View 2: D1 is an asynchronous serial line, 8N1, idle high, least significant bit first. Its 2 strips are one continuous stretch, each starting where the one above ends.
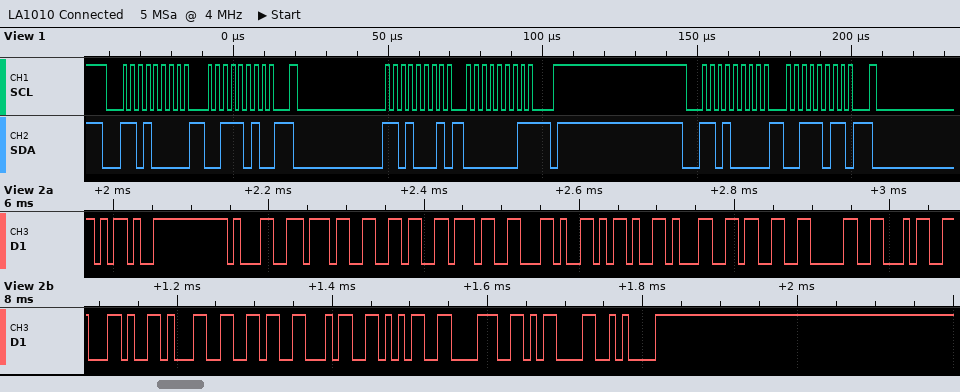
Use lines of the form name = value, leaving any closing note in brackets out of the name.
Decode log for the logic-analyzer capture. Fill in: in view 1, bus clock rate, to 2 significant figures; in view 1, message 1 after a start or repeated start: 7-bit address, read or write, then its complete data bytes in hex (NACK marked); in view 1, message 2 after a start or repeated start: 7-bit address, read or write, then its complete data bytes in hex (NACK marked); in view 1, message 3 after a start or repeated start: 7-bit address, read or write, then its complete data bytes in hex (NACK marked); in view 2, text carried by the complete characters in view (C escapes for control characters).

in view 1, bus clock rate, to 2 significant figures = 400 kHz
in view 1, message 1 after a start or repeated start: 7-bit address, read or write, then its complete data bytes in hex = 0x68 write: 3A
in view 1, message 2 after a start or repeated start: 7-bit address, read or write, then its complete data bytes in hex = 0x68 read: 01 NACK
in view 1, message 3 after a start or repeated start: 7-bit address, read or write, then its complete data bytes in hex = 0x68 write: 3B
in view 2, text carried by the complete characters in view = "-1767,-1304,16458\r\n"
